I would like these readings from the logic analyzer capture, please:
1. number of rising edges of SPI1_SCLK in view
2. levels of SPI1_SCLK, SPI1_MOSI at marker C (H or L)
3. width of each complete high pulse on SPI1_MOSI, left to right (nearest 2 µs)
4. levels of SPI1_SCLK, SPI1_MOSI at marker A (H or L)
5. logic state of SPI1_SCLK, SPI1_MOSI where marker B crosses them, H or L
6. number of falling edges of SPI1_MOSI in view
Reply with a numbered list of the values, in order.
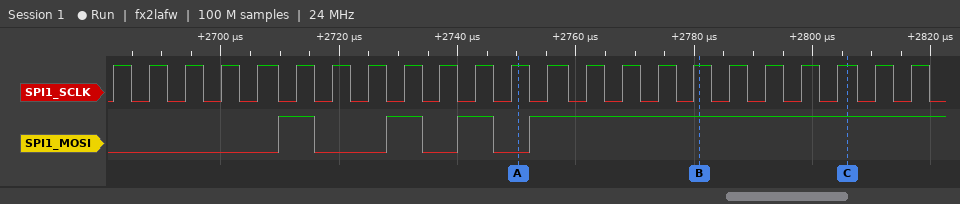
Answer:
1. 23
2. SPI1_SCLK=H, SPI1_MOSI=H
3. 6 µs, 6 µs, 6 µs
4. SPI1_SCLK=H, SPI1_MOSI=L
5. SPI1_SCLK=H, SPI1_MOSI=H
6. 3
